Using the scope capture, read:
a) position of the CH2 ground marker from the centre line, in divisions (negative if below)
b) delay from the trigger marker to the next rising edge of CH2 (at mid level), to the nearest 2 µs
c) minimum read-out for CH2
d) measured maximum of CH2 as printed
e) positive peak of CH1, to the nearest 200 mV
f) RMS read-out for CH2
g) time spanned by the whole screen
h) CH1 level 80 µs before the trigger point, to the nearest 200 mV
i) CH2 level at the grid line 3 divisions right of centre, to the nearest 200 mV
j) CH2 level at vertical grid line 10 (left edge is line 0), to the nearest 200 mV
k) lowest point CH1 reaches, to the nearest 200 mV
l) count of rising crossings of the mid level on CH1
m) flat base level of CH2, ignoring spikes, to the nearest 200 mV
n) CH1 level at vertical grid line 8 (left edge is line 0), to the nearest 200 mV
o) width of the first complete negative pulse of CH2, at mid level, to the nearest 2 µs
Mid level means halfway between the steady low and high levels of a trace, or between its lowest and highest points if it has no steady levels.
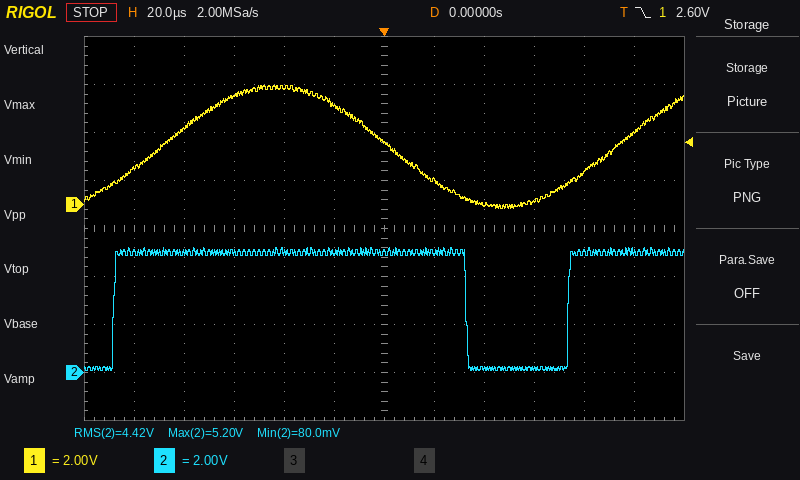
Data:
-3.0 div
74 µs
80.0 mV
5.20 V
5.0 V
4.42 V
240 µs
3.2 V
200 mV
5.0 V
-200 mV
2
200 mV
0.0 V
40 µs
